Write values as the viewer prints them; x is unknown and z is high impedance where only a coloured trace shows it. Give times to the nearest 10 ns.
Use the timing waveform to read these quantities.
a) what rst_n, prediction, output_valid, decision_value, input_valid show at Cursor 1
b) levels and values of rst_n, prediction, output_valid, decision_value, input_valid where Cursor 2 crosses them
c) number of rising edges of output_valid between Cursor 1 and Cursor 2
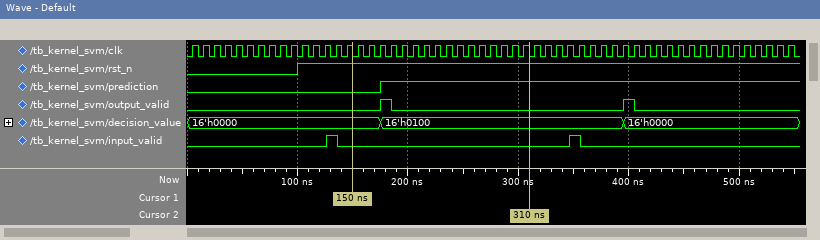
rst_n=1, prediction=0, output_valid=0, decision_value=16'h0000, input_valid=0
rst_n=1, prediction=1, output_valid=0, decision_value=16'h0100, input_valid=0
1
